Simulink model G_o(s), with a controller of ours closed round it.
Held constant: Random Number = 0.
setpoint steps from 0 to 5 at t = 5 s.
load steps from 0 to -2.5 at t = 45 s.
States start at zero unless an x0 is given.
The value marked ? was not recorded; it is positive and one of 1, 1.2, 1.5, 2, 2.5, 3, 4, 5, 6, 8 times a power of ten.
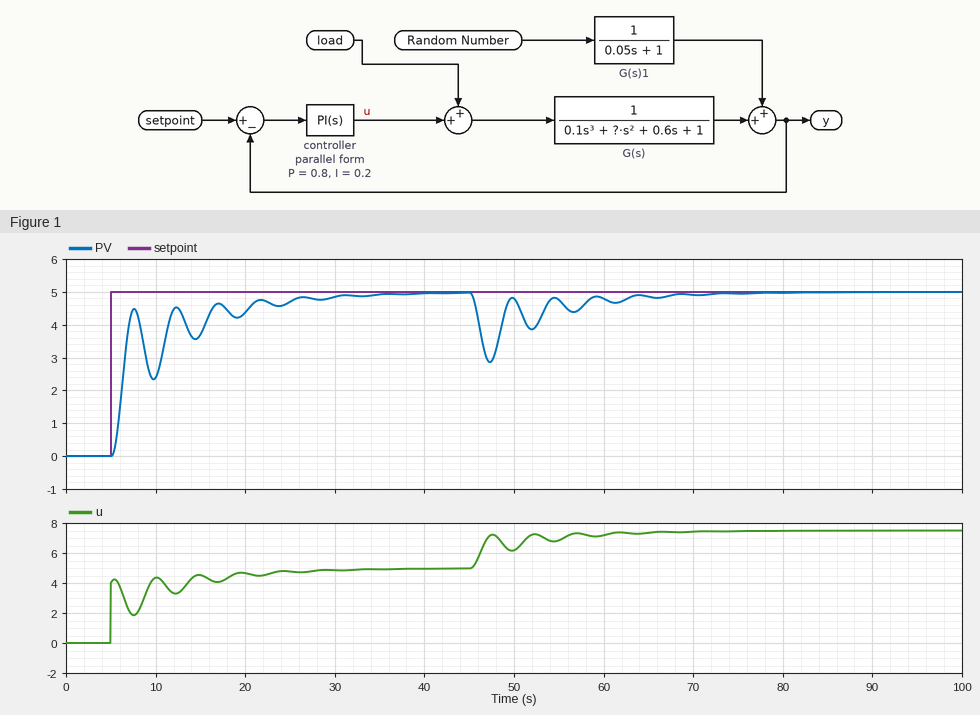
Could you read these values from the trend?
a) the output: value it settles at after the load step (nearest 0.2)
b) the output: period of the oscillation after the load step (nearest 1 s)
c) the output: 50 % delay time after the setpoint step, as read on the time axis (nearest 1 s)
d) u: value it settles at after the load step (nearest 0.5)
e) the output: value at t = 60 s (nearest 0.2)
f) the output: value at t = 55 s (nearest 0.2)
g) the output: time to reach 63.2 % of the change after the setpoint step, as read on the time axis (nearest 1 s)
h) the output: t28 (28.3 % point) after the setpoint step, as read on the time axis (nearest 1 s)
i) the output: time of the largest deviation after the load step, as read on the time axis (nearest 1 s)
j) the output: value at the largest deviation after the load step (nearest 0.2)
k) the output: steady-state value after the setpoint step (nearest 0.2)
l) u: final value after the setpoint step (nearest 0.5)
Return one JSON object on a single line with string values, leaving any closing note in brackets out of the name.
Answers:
{"the output: value it settles at after the load step": "5.0", "the output: period of the oscillation after the load step": "5 s", "the output: 50 % delay time after the setpoint step, as read on the time axis": "6 s", "u: value it settles at after the load step": "7.5", "the output: value at t = 60 s": "4.8", "the output: value at t = 55 s": "4.8", "the output: time to reach 63.2 % of the change after the setpoint step, as read on the time axis": "7 s", "the output: t28 (28.3 % point) after the setpoint step, as read on the time axis": "6 s", "the output: time of the largest deviation after the load step, as read on the time axis": "47 s", "the output: value at the largest deviation after the load step": "2.8", "the output: steady-state value after the setpoint step": "5.0", "u: final value after the setpoint step": "5.0"}
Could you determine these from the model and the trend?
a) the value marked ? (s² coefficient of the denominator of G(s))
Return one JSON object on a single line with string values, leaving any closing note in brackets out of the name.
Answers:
{"the value marked ? (s² coefficient of the denominator of G(s))": "1"}
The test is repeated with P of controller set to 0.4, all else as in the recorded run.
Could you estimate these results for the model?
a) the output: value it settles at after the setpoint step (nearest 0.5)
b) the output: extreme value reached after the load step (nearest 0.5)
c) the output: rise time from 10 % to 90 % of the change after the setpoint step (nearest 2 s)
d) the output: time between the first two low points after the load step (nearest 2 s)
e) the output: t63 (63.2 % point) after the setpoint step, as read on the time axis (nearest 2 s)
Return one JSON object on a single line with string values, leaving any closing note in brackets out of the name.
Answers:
{"the output: value it settles at after the setpoint step": "5.0", "the output: extreme value reached after the load step": "2.5", "the output: rise time from 10 % to 90 % of the change after the setpoint step": "12 s", "the output: time between the first two low points after the load step": "6 s", "the output: t63 (63.2 % point) after the setpoint step, as read on the time axis": "8 s"}
